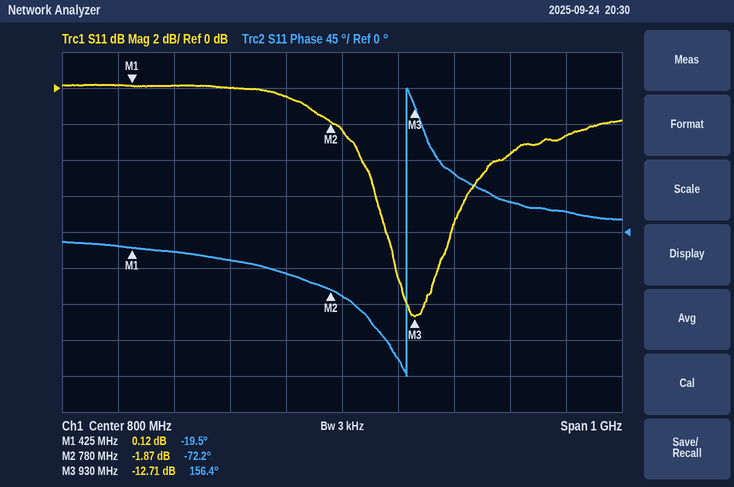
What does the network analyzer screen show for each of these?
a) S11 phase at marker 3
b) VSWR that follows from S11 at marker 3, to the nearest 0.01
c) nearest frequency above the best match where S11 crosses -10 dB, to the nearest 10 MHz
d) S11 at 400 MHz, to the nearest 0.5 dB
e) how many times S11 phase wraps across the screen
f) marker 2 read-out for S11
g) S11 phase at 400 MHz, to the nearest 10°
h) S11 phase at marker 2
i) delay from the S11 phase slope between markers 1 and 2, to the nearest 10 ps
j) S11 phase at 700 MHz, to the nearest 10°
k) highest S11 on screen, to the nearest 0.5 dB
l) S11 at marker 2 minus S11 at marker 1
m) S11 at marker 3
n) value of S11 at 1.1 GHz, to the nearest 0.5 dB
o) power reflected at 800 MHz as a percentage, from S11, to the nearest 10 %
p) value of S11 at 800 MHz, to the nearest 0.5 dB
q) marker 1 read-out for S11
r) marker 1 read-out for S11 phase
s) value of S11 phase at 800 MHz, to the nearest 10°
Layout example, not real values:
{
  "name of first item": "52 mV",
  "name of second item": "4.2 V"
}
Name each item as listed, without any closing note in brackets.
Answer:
{
  "S11 phase at marker 3": "156.4°",
  "VSWR that follows from S11 at marker 3, to the nearest 0.01": "1.60",
  "nearest frequency above the best match where S11 crosses -10 dB, to the nearest 10 MHz": "970 MHz",
  "S11 at 400 MHz, to the nearest 0.5 dB": "0.0 dB",
  "how many times S11 phase wraps across the screen": "1",
  "marker 2 read-out for S11": "-1.87 dB",
  "S11 phase at 400 MHz, to the nearest 10°": "-20°",
  "S11 phase at marker 2": "-72.2°",
  "delay from the S11 phase slope between markers 1 and 2, to the nearest 10 ps": "410 ps",
  "S11 phase at 700 MHz, to the nearest 10°": "-50°",
  "highest S11 on screen, to the nearest 0.5 dB": "0.0 dB",
  "S11 at marker 2 minus S11 at marker 1": "-1.99 dB",
  "S11 at marker 3": "-12.71 dB",
  "value of S11 at 1.1 GHz, to the nearest 0.5 dB": "-3.5 dB",
  "power reflected at 800 MHz as a percentage, from S11, to the nearest 10 %": "60 %",
  "value of S11 at 800 MHz, to the nearest 0.5 dB": "-2.5 dB",
  "marker 1 read-out for S11": "0.12 dB",
  "marker 1 read-out for S11 phase": "-19.5°",
  "value of S11 phase at 800 MHz, to the nearest 10°": "-80°"
}
